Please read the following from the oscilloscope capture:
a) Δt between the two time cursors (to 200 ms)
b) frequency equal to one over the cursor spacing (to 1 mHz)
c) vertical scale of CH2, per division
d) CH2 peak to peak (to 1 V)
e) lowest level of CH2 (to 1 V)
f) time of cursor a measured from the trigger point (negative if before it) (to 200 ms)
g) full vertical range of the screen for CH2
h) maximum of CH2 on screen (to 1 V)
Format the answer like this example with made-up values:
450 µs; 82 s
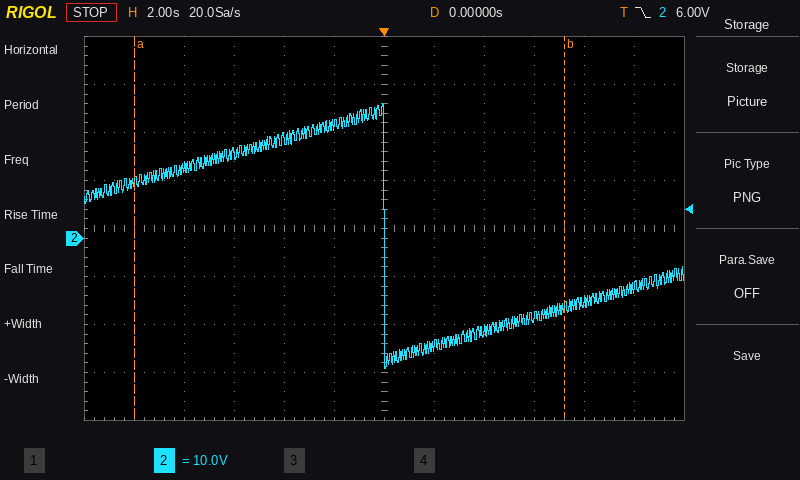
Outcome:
17.2 s; 58 mHz; 10 V; 55 V; -27 V; -10.0 s; 80 V; 28 V
